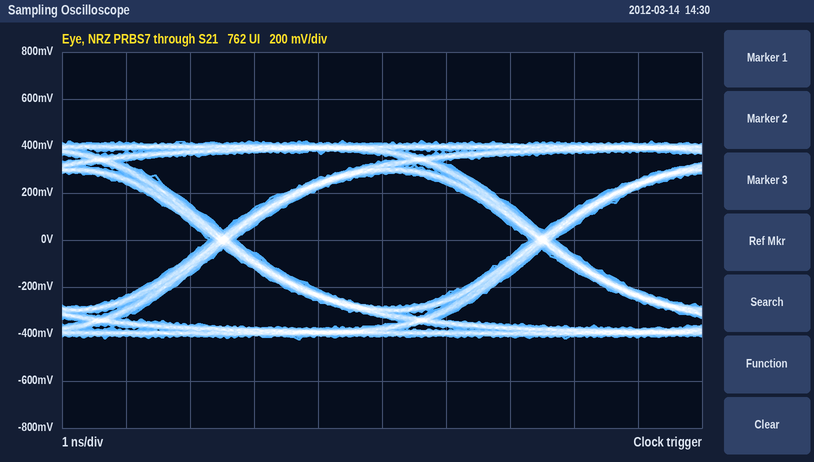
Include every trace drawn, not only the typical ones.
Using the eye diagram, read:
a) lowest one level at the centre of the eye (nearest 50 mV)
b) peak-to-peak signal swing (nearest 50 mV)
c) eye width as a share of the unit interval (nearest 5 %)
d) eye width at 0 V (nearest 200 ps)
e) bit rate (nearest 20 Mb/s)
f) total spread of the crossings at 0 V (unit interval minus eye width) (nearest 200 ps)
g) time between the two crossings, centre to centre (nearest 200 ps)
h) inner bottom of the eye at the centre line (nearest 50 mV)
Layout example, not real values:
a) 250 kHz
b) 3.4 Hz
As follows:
a) 300 mV
b) 850 mV
c) 90 %
d) 4.6 ns
e) 200 Mb/s
f) 400 ps
g) 5.0 ns
h) -300 mV
